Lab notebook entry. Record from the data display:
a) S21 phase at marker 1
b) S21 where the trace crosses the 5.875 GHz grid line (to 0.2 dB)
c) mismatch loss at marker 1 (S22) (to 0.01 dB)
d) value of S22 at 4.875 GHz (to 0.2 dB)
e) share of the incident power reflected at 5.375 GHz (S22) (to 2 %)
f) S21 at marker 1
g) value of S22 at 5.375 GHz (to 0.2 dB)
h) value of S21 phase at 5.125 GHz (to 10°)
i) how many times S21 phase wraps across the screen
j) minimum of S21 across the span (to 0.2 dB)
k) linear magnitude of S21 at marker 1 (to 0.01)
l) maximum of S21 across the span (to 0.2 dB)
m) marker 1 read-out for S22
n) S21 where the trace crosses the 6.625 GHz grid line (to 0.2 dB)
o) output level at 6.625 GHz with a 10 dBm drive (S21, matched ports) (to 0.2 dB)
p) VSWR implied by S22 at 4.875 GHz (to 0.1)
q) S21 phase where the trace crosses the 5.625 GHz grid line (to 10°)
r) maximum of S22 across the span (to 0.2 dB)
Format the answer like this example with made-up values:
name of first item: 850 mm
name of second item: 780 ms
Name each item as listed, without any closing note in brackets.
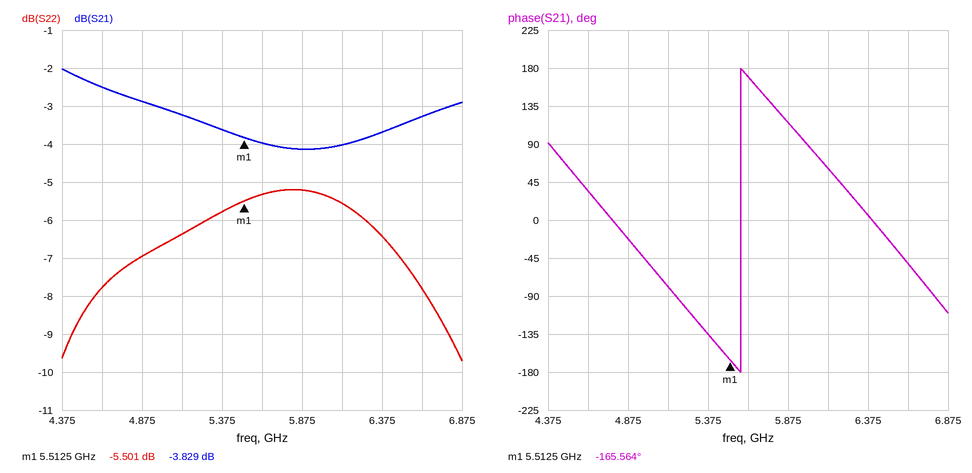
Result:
S21 phase at marker 1: -165.564°
S21 where the trace crosses the 5.875 GHz grid line: -4.2 dB
mismatch loss at marker 1 (S22): 1.44 dB
value of S22 at 4.875 GHz: -7.0 dB
share of the incident power reflected at 5.375 GHz (S22): 26 %
S21 at marker 1: -3.829 dB
value of S22 at 5.375 GHz: -5.8 dB
value of S21 phase at 5.125 GHz: -80°
how many times S21 phase wraps across the screen: 1
minimum of S21 across the span: -4.2 dB
linear magnitude of S21 at marker 1: 0.64
maximum of S21 across the span: -2.0 dB
marker 1 read-out for S22: -5.501 dB
S21 where the trace crosses the 6.625 GHz grid line: -3.2 dB
output level at 6.625 GHz with a 10 dBm drive (S21, matched ports): 6.8 dBm
VSWR implied by S22 at 4.875 GHz: 2.6
S21 phase where the trace crosses the 5.625 GHz grid line: 170°
maximum of S22 across the span: -5.2 dB
